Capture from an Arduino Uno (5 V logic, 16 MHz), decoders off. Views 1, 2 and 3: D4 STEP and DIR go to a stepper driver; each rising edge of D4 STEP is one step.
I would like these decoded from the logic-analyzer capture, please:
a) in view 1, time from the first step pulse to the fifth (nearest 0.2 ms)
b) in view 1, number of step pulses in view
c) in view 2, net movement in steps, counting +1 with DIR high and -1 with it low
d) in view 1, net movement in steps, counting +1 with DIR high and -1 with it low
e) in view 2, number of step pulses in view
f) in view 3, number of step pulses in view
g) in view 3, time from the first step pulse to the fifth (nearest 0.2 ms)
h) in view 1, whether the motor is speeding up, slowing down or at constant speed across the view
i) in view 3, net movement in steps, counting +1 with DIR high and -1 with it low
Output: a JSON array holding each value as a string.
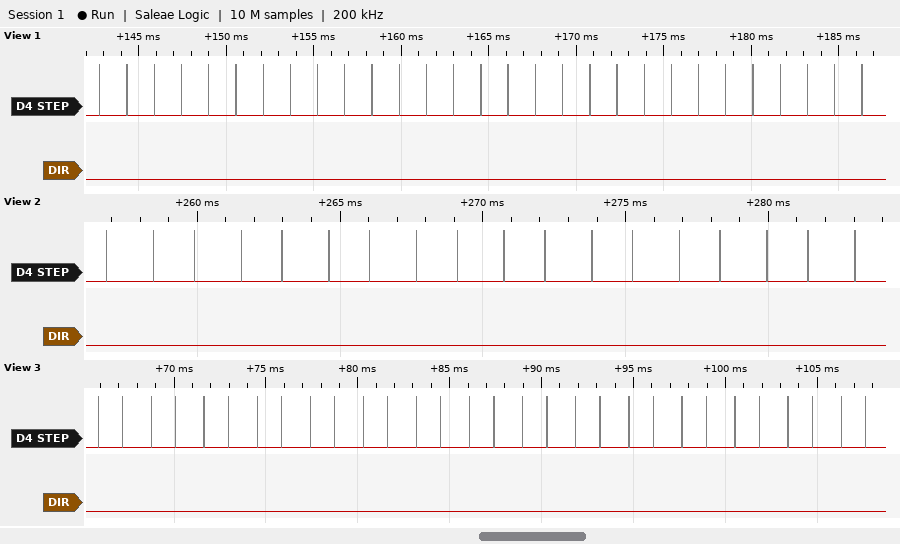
["6.2 ms", "29", "-18", "-29", "18", "30", "5.8 ms", "constant speed", "-30"]
